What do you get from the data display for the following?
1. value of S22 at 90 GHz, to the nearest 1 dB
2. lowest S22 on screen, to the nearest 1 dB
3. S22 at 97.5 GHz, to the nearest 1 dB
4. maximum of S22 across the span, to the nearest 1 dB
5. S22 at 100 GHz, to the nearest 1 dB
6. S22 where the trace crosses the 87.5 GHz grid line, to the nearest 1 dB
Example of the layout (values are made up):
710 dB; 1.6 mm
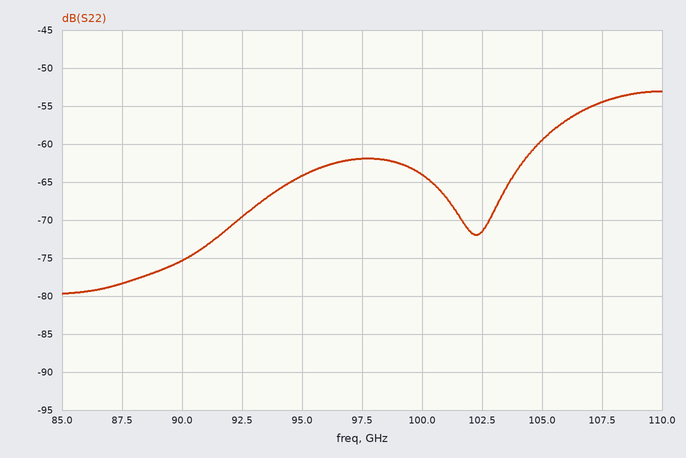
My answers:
-75 dB; -80 dB; -62 dB; -53 dB; -64 dB; -78 dB
